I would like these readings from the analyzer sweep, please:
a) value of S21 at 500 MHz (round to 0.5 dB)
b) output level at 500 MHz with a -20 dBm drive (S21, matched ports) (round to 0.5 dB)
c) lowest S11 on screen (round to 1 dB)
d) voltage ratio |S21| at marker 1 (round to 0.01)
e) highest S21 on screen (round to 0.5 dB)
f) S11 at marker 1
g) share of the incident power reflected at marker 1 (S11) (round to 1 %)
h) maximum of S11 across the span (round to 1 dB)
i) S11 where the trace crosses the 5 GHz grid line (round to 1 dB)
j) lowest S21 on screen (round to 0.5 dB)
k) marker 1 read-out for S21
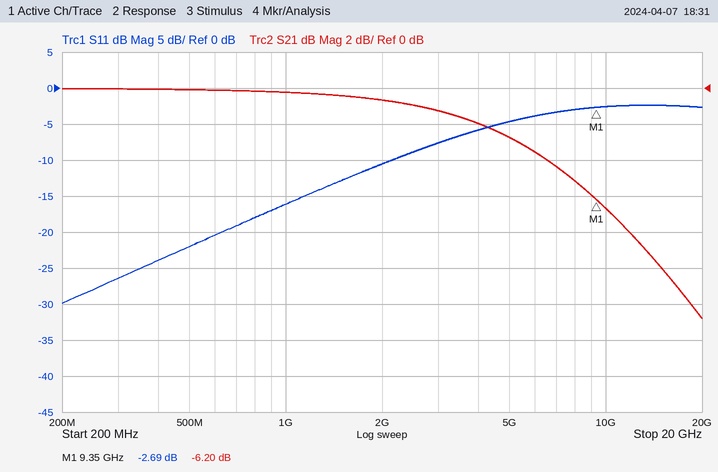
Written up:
0.0 dB
-20.0 dBm
-30 dB
0.49
0.0 dB
-2.69 dB
54 %
-2 dB
-5 dB
-13.0 dB
-6.20 dB
